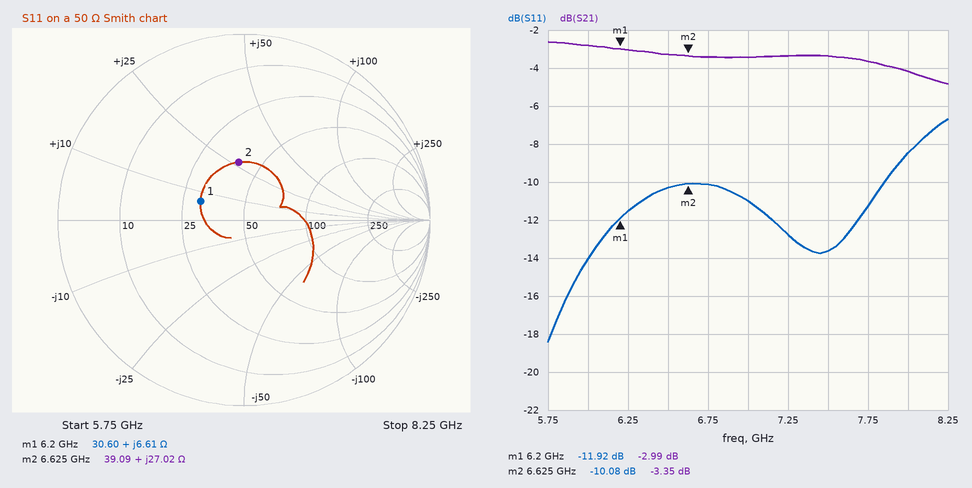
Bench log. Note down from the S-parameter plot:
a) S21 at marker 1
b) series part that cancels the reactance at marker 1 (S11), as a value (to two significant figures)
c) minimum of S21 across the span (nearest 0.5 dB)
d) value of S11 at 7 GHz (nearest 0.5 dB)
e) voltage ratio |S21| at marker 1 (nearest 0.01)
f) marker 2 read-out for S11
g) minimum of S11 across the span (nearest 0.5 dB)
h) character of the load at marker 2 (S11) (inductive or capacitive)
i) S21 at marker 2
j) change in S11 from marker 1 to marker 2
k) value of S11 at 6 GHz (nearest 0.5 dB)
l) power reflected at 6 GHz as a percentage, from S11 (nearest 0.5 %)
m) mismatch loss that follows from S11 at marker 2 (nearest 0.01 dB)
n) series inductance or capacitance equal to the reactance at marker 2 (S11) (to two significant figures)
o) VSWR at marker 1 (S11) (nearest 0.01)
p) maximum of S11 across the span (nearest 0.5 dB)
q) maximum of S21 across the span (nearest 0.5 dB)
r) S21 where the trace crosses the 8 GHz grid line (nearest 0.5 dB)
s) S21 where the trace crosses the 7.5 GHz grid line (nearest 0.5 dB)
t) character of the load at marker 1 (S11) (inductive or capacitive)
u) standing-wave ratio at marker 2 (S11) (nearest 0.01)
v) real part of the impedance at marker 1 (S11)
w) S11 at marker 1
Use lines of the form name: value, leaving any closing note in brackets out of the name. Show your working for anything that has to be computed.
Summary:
S21 at marker 1: -2.99 dB
series part that cancels the reactance at marker 1 (S11), as a value: C = 1/(2π × 6.2 GHz × 6.61 Ω) ≈ 3.9 pF
minimum of S21 across the span: -5.0 dB
value of S11 at 7 GHz: -11.0 dB
voltage ratio |S21| at marker 1: 10^(-2.99/20) ≈ 0.71
marker 2 read-out for S11: -10.08 dB
minimum of S11 across the span: -18.5 dB
character of the load at marker 2 (S11): inductive
S21 at marker 2: -3.35 dB
change in S11 from marker 1 to marker 2: -10.08 − (-11.92) = 1.84 dB
value of S11 at 6 GHz: -14.0 dB
power reflected at 6 GHz as a percentage, from S11: 10^(-14/10) ≈ 4.0 %
mismatch loss that follows from S11 at marker 2: −10 log10(1 − 10^(-10.08/10)) ≈ 0.45 dB
series inductance or capacitance equal to the reactance at marker 2 (S11): L = 27.02 Ω/(2π × 6.625 GHz) ≈ 649 pH, so 650 pH to two significant figures
VSWR at marker 1 (S11): 1.68
maximum of S11 across the span: -6.5 dB
maximum of S21 across the span: -2.5 dB
S21 where the trace crosses the 8 GHz grid line: -4.0 dB
S21 where the trace crosses the 7.5 GHz grid line: -3.5 dB
character of the load at marker 1 (S11): inductive
standing-wave ratio at marker 2 (S11): 1.91
real part of the impedance at marker 1: 30.60 Ω
S11 at marker 1: -11.92 dB
